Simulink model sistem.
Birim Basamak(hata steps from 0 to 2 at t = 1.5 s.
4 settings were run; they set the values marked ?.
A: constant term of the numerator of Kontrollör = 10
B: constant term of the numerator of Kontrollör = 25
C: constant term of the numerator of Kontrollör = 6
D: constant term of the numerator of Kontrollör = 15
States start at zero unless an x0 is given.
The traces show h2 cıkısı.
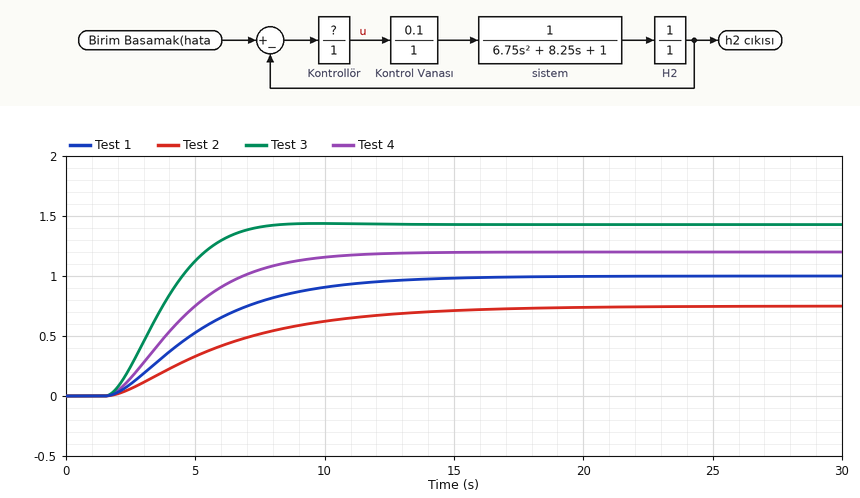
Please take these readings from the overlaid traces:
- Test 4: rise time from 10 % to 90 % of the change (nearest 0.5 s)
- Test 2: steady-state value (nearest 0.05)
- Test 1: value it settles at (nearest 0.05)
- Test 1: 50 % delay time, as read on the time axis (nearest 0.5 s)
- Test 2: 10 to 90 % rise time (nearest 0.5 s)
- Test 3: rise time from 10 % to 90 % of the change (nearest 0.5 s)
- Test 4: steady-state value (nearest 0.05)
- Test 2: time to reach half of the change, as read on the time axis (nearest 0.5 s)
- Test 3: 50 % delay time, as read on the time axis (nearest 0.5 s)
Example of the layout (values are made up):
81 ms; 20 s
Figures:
5.5 s; 0.75; 1.00; 5.0 s; 9.5 s; 3.5 s; 1.20; 5.5 s; 3.5 s
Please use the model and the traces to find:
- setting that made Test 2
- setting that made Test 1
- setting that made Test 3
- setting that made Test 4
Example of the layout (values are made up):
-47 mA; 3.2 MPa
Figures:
C; A; B; D
